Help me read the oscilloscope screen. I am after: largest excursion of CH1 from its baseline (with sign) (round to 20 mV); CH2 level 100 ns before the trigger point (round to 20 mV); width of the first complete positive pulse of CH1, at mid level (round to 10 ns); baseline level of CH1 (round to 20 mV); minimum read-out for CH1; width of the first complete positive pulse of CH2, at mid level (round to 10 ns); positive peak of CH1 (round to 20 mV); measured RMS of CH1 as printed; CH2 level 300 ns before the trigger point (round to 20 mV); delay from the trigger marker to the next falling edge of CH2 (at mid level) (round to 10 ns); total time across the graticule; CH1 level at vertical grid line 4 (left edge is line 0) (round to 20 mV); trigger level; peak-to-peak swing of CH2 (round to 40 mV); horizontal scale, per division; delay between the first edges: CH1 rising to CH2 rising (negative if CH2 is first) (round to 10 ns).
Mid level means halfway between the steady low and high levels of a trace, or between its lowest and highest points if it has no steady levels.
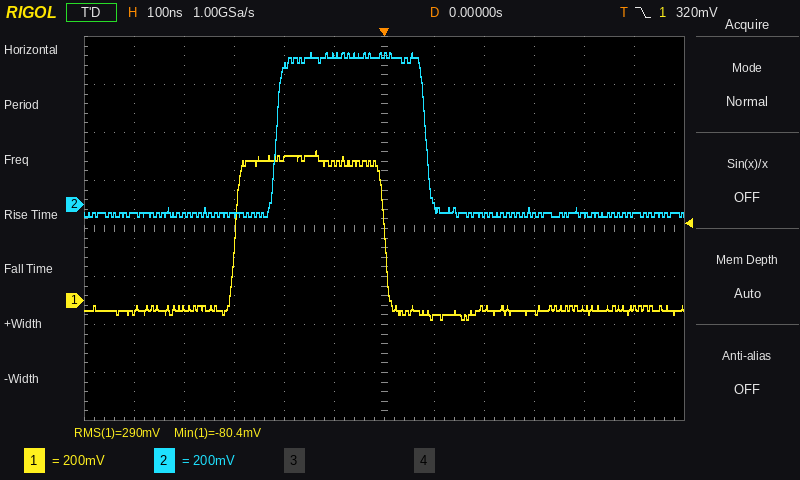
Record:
+660 mV
620 mV
300 ns
-40 mV
-80.4 mV
300 ns
620 mV
290 mV
-40 mV
80 ns
1.2 µs
600 mV
320 mV
680 mV
100 ns
+80 ns
